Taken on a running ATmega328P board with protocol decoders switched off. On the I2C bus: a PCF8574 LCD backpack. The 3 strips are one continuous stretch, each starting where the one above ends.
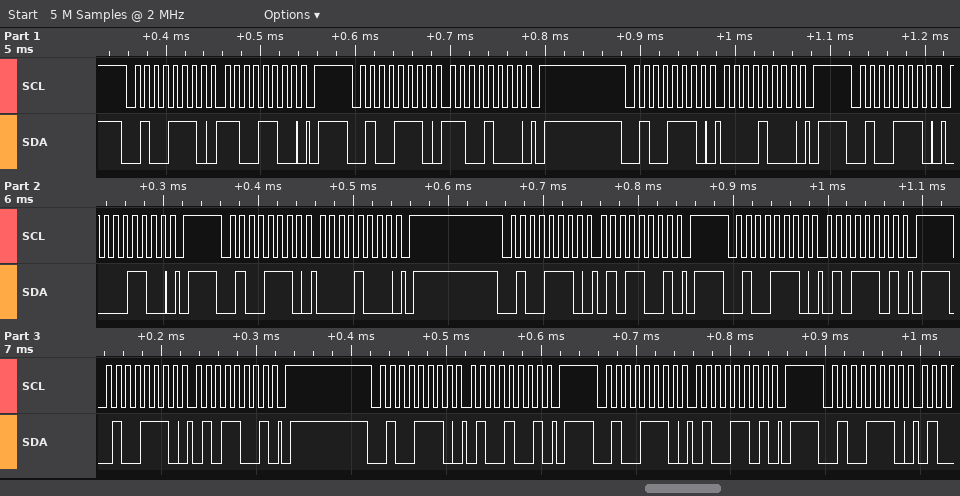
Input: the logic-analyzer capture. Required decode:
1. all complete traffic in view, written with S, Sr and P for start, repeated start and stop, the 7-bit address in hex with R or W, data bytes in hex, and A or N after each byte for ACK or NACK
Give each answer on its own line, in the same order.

S 27W A CC A P S 27W A C8 A P S 27W A 08 A P S 27W A 0C A P S 27W A 08 A P S 27W A 59 A P S 27W A 5D A P S 27W A 59 A P S 27W A 49 A P S 27W A 4D A P S 27W A
